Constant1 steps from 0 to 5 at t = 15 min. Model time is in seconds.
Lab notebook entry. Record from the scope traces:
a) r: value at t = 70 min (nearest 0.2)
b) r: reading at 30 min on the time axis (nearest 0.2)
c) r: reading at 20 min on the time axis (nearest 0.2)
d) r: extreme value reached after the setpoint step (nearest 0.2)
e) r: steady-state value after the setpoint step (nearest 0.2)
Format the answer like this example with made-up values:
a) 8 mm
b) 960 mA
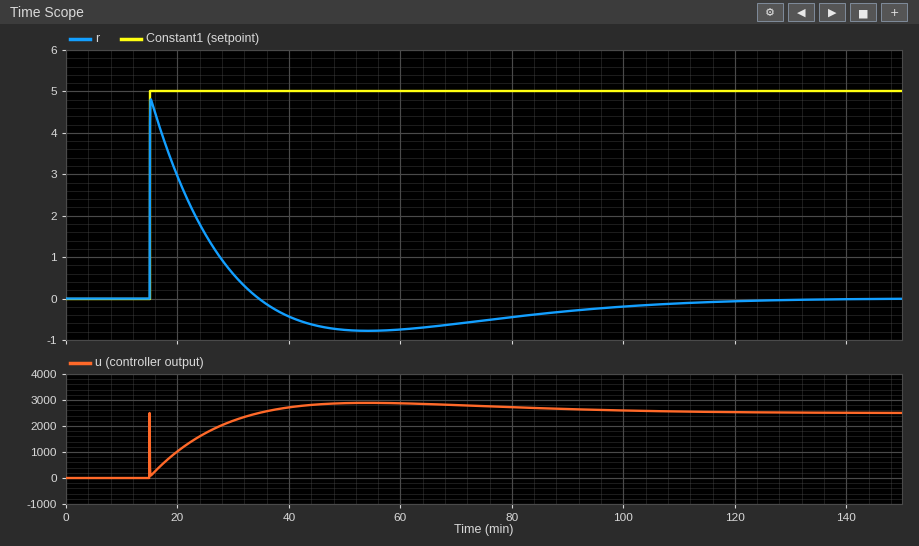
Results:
a) -0.6
b) 0.6
c) 3.0
d) 4.8
e) 0.0
